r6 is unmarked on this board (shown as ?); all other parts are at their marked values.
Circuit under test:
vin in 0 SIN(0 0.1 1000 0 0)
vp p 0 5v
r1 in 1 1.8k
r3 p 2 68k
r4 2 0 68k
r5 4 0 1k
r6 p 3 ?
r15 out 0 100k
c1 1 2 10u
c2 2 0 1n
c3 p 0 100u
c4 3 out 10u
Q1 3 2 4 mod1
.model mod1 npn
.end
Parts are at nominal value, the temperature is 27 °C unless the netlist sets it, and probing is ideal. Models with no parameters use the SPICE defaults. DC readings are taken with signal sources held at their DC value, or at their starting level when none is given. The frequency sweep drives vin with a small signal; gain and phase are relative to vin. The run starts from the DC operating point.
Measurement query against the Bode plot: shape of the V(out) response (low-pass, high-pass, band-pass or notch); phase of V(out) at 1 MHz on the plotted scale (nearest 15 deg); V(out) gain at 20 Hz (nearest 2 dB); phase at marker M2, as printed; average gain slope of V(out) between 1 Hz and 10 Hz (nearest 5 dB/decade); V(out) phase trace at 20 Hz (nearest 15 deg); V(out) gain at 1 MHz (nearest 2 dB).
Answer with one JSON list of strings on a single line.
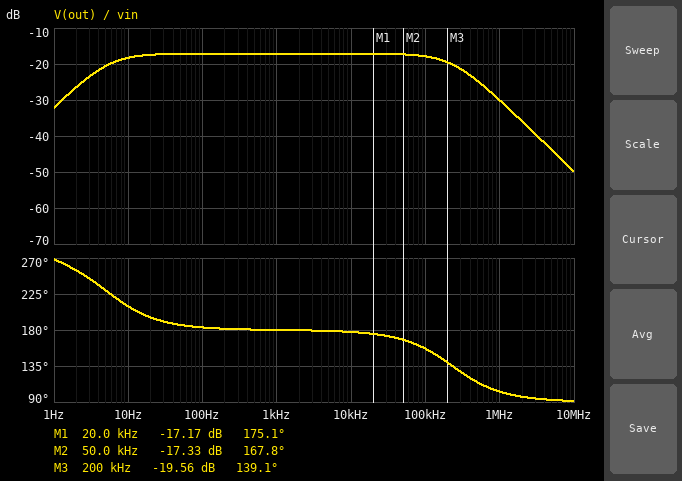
["band-pass", "105 deg", "-18 dB", "167.8 deg", "15 dB/decade", "195 deg", "-30 dB"]
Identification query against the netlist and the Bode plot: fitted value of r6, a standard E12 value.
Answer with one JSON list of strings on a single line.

["4.7 kΩ"]
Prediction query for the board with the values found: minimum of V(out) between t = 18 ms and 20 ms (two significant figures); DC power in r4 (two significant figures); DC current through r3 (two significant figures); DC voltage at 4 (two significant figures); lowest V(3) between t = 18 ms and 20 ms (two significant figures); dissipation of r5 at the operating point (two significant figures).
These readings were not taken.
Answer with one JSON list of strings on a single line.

["-2.5 mV", "40 µW", "49 µA", "880 mV", "980 mV", "770 µW"]
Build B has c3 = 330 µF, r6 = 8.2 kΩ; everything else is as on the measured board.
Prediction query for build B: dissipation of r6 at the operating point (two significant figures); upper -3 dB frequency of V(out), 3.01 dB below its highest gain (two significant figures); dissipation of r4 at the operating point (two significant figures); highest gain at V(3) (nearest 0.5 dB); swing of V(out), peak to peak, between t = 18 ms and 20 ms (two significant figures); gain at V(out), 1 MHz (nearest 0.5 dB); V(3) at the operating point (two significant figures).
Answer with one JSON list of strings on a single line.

["2.3 mW", "240 kHz", "26 µW", "-24.5 dB", "110 mV", "-37.0 dB", "640 mV"]
